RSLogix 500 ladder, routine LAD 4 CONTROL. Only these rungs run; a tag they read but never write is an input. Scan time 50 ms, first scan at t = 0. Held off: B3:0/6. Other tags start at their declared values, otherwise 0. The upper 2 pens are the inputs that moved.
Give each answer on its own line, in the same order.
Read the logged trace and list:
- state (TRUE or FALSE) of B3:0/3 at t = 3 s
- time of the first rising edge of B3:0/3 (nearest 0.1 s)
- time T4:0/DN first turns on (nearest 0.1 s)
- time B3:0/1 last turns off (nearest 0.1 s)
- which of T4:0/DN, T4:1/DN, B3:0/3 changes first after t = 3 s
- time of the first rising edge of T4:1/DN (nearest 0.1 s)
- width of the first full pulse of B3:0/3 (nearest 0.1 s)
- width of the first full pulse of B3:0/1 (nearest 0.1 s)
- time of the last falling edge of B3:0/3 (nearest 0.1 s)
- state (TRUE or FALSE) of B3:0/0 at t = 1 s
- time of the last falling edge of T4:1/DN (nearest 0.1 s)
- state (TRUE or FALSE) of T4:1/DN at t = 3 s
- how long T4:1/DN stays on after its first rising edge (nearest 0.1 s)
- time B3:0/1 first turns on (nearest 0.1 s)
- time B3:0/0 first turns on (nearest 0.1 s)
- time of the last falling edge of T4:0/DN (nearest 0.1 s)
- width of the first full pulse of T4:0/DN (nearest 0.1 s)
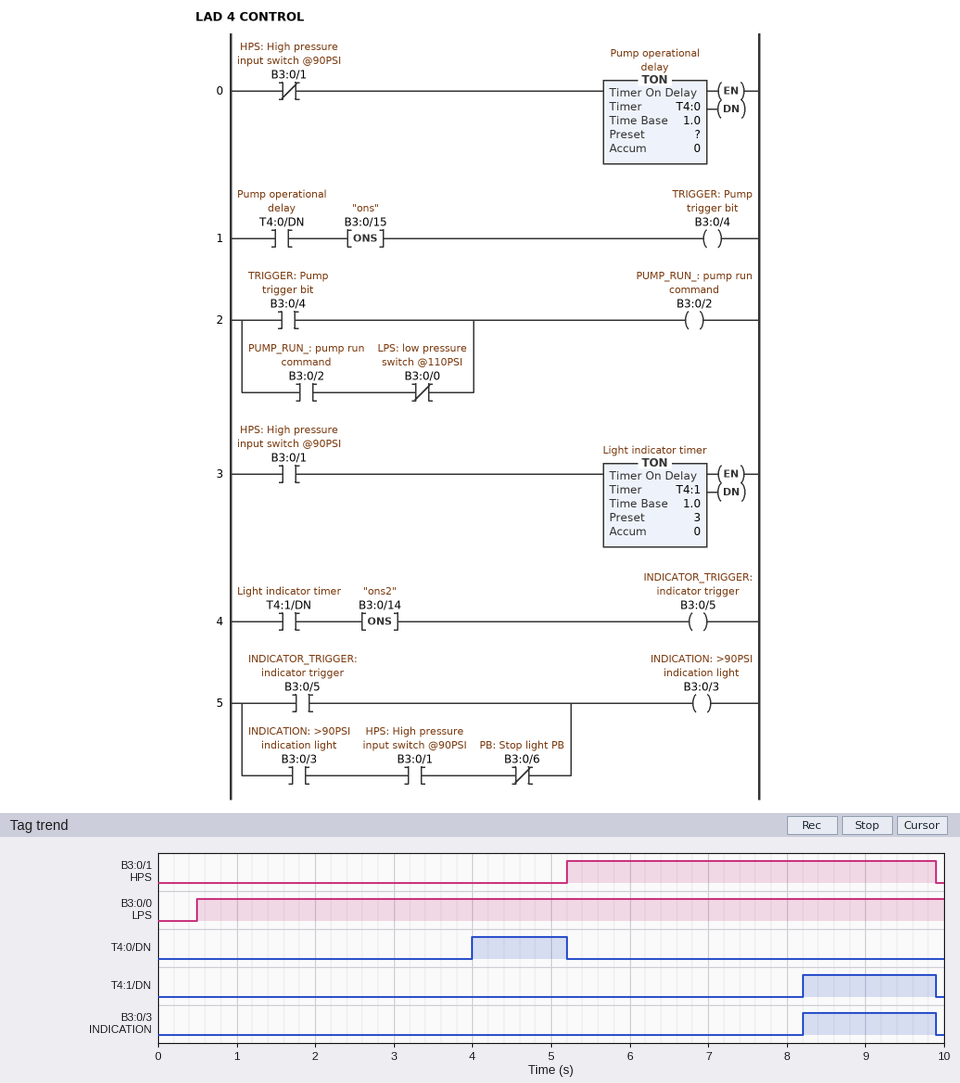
FALSE
8.2 s
4.0 s
9.9 s
T4:0/DN
8.2 s
1.7 s
4.7 s
9.9 s
TRUE
9.9 s
FALSE
1.7 s
5.2 s
0.5 s
5.2 s
1.2 s
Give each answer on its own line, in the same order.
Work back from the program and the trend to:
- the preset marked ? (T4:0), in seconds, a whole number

4 s
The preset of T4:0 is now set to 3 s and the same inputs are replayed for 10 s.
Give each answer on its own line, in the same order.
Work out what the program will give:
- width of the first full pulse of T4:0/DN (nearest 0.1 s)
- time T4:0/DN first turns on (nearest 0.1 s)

2.2 s
3.0 s
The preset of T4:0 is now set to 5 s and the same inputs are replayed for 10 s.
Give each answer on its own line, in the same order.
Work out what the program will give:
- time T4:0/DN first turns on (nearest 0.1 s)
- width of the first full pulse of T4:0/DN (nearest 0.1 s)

5.0 s
0.2 s
